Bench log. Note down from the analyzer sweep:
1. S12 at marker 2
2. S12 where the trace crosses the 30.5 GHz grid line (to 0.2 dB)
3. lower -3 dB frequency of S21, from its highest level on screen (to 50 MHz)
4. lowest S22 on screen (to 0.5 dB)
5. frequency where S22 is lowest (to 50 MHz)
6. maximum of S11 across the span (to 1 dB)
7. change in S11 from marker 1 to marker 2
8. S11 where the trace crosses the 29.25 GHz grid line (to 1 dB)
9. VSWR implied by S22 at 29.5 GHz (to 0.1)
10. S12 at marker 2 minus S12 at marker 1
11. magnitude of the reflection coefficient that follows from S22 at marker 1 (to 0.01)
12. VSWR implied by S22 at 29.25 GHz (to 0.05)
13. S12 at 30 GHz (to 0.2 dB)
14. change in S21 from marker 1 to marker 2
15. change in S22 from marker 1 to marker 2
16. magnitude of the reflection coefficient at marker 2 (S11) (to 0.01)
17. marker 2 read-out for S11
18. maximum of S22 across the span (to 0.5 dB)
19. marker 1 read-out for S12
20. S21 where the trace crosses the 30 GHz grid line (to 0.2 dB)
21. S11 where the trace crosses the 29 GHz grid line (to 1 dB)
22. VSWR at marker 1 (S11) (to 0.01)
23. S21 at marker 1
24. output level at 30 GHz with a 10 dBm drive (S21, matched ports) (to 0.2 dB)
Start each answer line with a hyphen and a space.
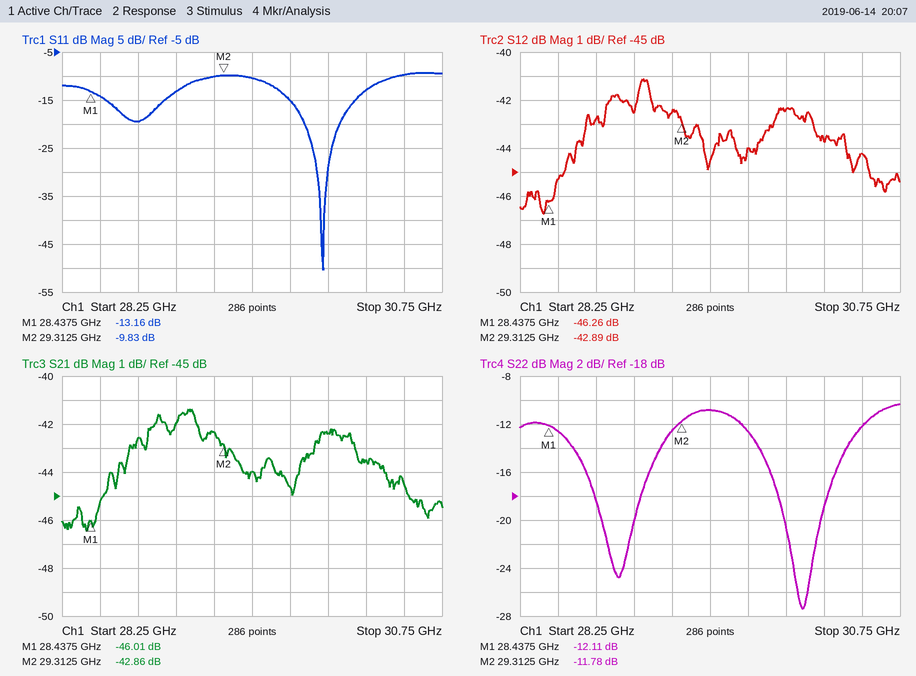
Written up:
- -42.89 dB
- -44.2 dB
- 28.60 GHz
- -27.5 dB
- 30.10 GHz
- -9 dB
- 3.33 dB
- -10 dB
- 1.8
- 3.37 dB
- 0.25
- 1.60
- -42.4 dB
- 3.15 dB
- 0.33 dB
- 0.32
- -9.83 dB
- -10.5 dB
- -46.26 dB
- -42.4 dB
- -13 dB
- 1.56
- -46.01 dB
- -32.4 dBm
